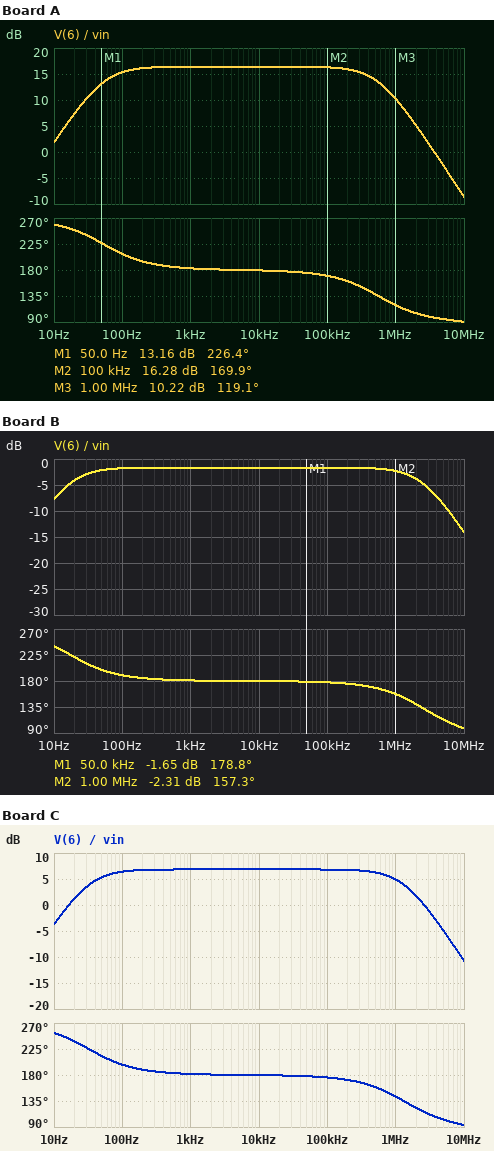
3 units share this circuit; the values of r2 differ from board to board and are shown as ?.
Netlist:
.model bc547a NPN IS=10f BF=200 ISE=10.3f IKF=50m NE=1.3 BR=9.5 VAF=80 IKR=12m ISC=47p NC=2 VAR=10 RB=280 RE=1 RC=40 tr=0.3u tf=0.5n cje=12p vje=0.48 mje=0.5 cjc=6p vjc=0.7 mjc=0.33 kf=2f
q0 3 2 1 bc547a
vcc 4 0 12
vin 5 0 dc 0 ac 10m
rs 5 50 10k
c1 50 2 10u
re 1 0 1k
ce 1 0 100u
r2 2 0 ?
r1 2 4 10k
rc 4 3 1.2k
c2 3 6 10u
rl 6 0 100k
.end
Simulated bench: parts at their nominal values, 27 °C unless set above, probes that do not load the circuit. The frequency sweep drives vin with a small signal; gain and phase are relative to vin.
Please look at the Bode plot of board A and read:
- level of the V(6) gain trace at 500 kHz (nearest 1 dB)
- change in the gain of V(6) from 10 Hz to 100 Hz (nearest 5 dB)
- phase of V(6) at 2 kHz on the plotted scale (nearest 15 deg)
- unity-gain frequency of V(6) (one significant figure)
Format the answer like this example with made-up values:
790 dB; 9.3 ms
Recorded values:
14 dB; 15 dB; 180 deg; 4 MHz
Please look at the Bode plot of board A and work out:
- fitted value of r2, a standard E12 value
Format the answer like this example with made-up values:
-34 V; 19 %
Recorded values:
2.7 kΩ
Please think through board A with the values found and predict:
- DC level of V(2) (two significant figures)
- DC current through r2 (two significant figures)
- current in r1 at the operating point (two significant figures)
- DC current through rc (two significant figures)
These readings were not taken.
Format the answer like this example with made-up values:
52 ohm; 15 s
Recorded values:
2.5 V; 930 µA; 950 µA; 1.8 mA
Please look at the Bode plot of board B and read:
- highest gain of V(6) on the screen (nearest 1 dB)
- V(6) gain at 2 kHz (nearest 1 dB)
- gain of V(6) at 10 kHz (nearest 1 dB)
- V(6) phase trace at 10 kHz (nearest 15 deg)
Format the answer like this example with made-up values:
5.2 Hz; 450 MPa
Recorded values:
-2 dB; -2 dB; -2 dB; 180 deg
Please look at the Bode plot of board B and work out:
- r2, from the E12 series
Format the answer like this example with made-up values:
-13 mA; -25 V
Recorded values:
820 Ω
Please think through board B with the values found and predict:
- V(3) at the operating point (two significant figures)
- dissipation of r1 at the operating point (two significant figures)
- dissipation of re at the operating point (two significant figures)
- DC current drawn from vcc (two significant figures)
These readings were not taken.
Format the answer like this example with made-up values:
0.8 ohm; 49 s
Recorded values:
12 V; 12 mW; 82 µW; 1.4 mA
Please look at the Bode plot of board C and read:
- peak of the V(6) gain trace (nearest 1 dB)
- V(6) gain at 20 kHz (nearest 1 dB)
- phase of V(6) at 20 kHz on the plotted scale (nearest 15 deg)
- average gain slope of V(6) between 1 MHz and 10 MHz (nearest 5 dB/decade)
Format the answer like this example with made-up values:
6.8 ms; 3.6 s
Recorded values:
7 dB; 7 dB; 180 deg; -15 dB/decade
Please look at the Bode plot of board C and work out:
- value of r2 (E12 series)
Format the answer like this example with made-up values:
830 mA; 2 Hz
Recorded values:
1.2 kΩ
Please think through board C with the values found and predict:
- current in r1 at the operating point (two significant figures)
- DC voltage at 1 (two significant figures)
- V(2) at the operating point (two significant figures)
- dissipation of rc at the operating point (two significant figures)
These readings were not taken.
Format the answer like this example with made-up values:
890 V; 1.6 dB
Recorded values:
1.1 mA; 640 mV; 1.3 V; 480 µW
